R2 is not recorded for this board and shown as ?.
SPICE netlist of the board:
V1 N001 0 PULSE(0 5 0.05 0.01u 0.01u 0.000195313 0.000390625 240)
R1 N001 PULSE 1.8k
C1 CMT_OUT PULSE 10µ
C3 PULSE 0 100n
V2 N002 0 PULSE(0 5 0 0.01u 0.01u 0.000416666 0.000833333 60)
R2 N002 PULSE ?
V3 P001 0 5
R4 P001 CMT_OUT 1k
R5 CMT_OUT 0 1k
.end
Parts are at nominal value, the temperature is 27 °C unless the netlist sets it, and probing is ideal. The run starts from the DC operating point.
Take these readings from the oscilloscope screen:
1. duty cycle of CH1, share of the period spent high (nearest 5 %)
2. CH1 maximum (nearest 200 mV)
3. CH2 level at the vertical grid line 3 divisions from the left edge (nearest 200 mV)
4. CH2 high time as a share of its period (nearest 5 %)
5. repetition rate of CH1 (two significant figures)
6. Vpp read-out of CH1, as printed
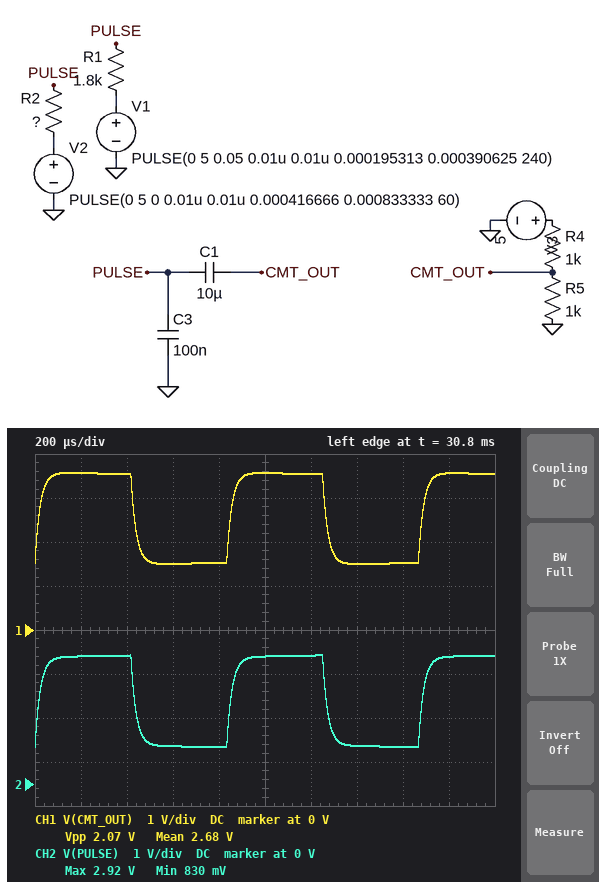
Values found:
50 %
3.6 V
800 mV
50 %
1.2 kHz
2.07 V
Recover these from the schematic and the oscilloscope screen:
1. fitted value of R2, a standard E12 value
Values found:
560 Ω
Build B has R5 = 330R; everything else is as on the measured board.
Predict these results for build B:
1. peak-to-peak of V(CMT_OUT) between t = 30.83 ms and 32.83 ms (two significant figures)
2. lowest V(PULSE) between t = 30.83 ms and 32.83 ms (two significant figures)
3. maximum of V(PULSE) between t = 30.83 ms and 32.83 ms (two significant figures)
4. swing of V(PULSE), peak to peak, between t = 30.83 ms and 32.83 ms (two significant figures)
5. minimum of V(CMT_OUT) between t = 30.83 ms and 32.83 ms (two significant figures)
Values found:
1.4 V
1.2 V
2.6 V
1.5 V
540 mV
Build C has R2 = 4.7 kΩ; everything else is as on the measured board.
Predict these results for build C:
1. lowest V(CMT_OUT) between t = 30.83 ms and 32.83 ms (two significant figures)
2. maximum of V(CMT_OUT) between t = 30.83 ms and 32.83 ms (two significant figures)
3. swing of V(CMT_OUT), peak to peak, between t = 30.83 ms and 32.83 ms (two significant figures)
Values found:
2.3 V
2.7 V
380 mV
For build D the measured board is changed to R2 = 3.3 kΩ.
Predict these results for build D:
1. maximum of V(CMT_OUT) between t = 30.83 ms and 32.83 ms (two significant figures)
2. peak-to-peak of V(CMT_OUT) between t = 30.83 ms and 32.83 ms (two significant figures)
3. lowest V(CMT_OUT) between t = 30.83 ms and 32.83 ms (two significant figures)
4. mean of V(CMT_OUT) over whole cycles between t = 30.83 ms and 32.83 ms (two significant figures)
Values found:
2.8 V
530 mV
2.3 V
2.5 V
